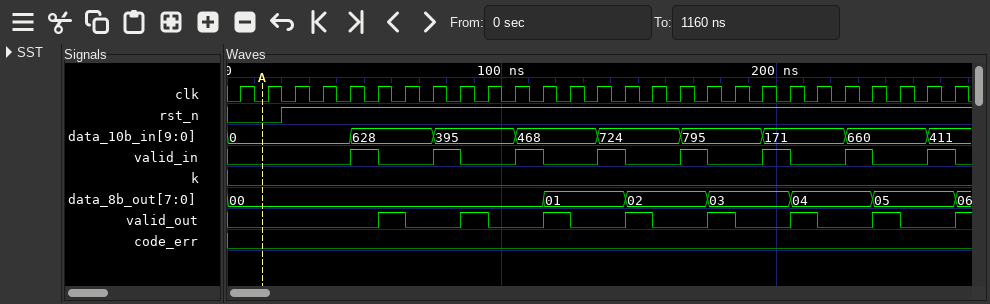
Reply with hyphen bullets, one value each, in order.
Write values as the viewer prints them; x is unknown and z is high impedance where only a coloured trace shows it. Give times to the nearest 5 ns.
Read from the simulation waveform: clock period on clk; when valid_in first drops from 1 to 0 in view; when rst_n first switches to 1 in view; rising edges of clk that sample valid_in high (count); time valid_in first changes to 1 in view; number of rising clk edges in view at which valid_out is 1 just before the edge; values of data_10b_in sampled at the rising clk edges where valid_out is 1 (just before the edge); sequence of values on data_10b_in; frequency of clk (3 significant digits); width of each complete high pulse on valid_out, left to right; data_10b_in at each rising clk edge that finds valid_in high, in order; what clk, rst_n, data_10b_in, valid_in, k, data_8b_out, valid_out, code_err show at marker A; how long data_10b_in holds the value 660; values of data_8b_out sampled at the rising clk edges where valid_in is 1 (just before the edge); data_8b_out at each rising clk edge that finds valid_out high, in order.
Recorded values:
- 10 ns
- 55 ns
- 20 ns
- 8
- 45 ns
- 7
- 628, 395, 468, 724, 795, 171, 660
- 0, 628, 395, 468, 724, 795, 171, 660, 411
- 100 MHz
- 10 ns, 10 ns, 10 ns, 10 ns, 10 ns, 10 ns, 10 ns
- 628, 395, 468, 724, 795, 171, 660, 411
- clk=0, rst_n=0, data_10b_in=0, valid_in=0, k=0, data_8b_out=00, valid_out=0, code_err=0
- 30 ns
- 00, 00, 00, 01, 02, 03, 04, 05
- 00, 00, 01, 02, 03, 04, 05
